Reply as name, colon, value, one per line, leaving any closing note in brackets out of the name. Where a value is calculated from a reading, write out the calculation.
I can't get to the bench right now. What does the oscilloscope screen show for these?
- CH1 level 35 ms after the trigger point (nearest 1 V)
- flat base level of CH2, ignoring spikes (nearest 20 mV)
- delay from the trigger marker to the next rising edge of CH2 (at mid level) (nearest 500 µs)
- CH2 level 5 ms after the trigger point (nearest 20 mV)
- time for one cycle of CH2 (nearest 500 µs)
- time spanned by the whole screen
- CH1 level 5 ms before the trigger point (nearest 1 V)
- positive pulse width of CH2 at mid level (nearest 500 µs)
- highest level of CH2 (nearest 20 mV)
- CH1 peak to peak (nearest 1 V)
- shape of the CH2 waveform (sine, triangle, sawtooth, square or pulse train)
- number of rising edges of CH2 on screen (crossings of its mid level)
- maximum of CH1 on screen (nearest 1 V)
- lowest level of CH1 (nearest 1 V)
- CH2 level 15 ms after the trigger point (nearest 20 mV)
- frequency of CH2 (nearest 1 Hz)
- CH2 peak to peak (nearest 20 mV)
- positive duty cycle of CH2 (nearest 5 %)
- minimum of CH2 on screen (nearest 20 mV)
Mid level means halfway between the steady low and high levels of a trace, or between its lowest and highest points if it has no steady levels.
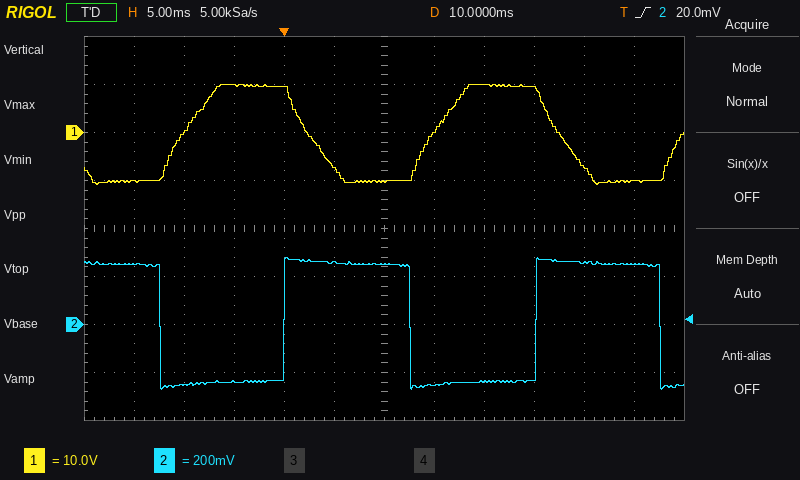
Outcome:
CH1 level 35 ms after the trigger point: -10 V
flat base level of CH2, ignoring spikes: -240 mV
delay from the trigger marker to the next rising edge of CH2 (at mid level): 25.0 ms
CH2 level 5 ms after the trigger point: 260 mV
time for one cycle of CH2: 25.0 ms
time spanned by the whole screen: 60 ms
CH1 level 5 ms before the trigger point: 10 V
positive pulse width of CH2 at mid level: 12.5 ms
highest level of CH2: 280 mV
CH1 peak to peak: 10 V − (-11 V) = 21 V
shape of the CH2 waveform: square
number of rising edges of CH2 on screen: 2
maximum of CH1 on screen: 10 V
lowest level of CH1: -11 V
CH2 level 15 ms after the trigger point: -260 mV
frequency of CH2: 1 / 25.0 ms ≈ 40 Hz
CH2 peak to peak: 280 mV − (-280 mV) = 560 mV
positive duty cycle of CH2: 12.5 ms / 25.0 ms ≈ 50 %
minimum of CH2 on screen: -280 mV
